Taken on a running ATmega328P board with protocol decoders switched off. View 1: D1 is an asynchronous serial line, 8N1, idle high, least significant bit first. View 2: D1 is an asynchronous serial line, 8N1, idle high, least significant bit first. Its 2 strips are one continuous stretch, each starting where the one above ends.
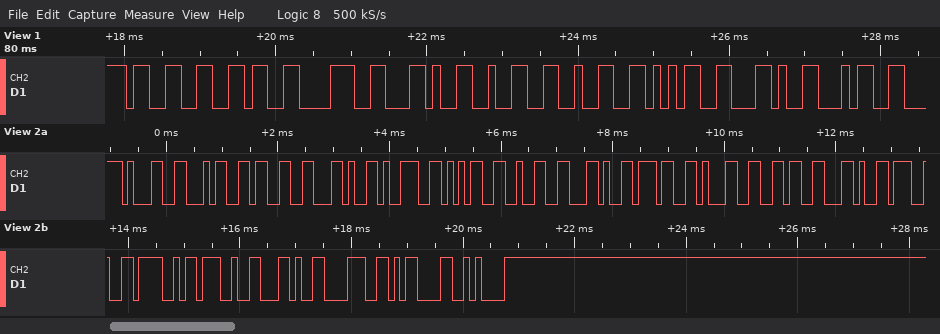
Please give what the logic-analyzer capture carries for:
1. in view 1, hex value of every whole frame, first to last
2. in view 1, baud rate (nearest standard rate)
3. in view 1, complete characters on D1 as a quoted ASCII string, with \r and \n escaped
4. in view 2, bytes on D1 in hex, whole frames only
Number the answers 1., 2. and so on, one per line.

1. 0x33 0x36 0x38 0x2C 0x32 0x32 0x35 0x2C 0x34
2. 9600 baud
3. "368,225,4"
4. 0x31 0x34 0x33 0x2C 0x39 0x35 0x32 0x2C 0x37 0x31 0x36 0x2C 0x27 0x4F 0x27 0x2C 0x38 0x0D 0x0A
